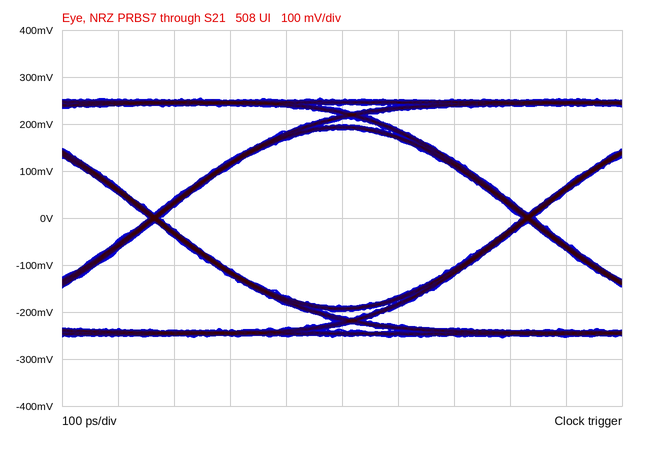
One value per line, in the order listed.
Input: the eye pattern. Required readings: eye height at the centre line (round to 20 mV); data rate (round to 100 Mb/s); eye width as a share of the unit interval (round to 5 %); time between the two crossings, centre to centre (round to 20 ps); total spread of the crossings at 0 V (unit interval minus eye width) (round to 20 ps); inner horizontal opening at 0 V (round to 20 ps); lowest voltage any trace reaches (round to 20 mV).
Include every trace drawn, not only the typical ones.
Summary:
380 mV
1.5 Gb/s
95 %
660 ps
20 ps
640 ps
-260 mV
